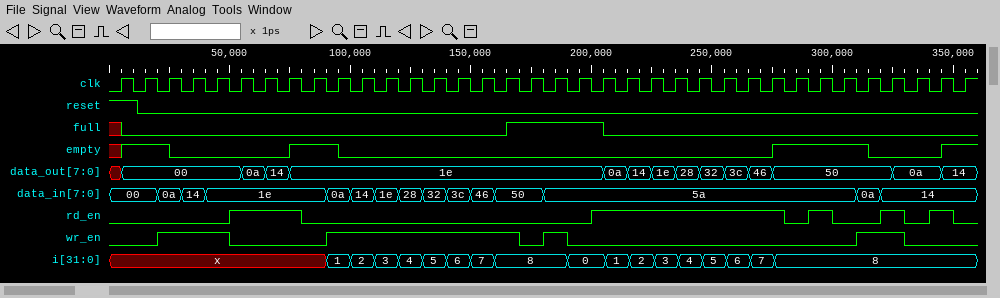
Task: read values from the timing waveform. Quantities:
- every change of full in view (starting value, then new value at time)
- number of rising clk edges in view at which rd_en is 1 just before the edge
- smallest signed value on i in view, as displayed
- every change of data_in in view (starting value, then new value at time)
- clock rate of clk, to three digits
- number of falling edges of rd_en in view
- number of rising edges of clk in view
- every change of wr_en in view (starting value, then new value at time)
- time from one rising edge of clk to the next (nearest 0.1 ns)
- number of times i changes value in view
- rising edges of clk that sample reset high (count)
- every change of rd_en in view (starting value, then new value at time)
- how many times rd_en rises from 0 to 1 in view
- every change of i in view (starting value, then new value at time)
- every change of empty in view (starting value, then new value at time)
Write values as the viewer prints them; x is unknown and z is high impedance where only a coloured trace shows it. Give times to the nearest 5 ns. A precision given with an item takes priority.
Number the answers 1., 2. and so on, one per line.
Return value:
1. x, 0 at 5 ns, 1 at 165 ns, 0 at 205 ns
2. 14
3. 0
4. 00, 0a at 20 ns, 14 at 30 ns, 1e at 40 ns, 0a at 90 ns, 14 at 100 ns, 1e at 110 ns, 28 at 120 ns, 32 at 130 ns, 3c at 140 ns, 46 at 150 ns, 50 at 160 ns, 5a at 180 ns, 0a at 310 ns, 14 at 320 ns
5. 100 MHz
6. 5
7. 36
8. 0, 1 at 20 ns, 0 at 50 ns, 1 at 90 ns, 0 at 170 ns, 1 at 180 ns, 0 at 190 ns, 1 at 310 ns, 0 at 330 ns
9. 10 ns
10. 17
11. 1
12. 0, 1 at 50 ns, 0 at 80 ns, 1 at 200 ns, 0 at 280 ns, 1 at 290 ns, 0 at 300 ns, 1 at 320 ns, 0 at 330 ns, 1 at 340 ns, 0 at 350 ns
13. 5
14. x, 1 at 90 ns, 2 at 100 ns, 3 at 110 ns, 4 at 120 ns, 5 at 130 ns, 6 at 140 ns, 7 at 150 ns, 8 at 160 ns, 0 at 190 ns, 1 at 205 ns, 2 at 215 ns, 3 at 225 ns, 4 at 235 ns, 5 at 245 ns, 6 at 255 ns, 7 at 265 ns, 8 at 275 ns
15. x, 1 at 5 ns, 0 at 25 ns, 1 at 75 ns, 0 at 95 ns, 1 at 275 ns, 0 at 315 ns, 1 at 345 ns
